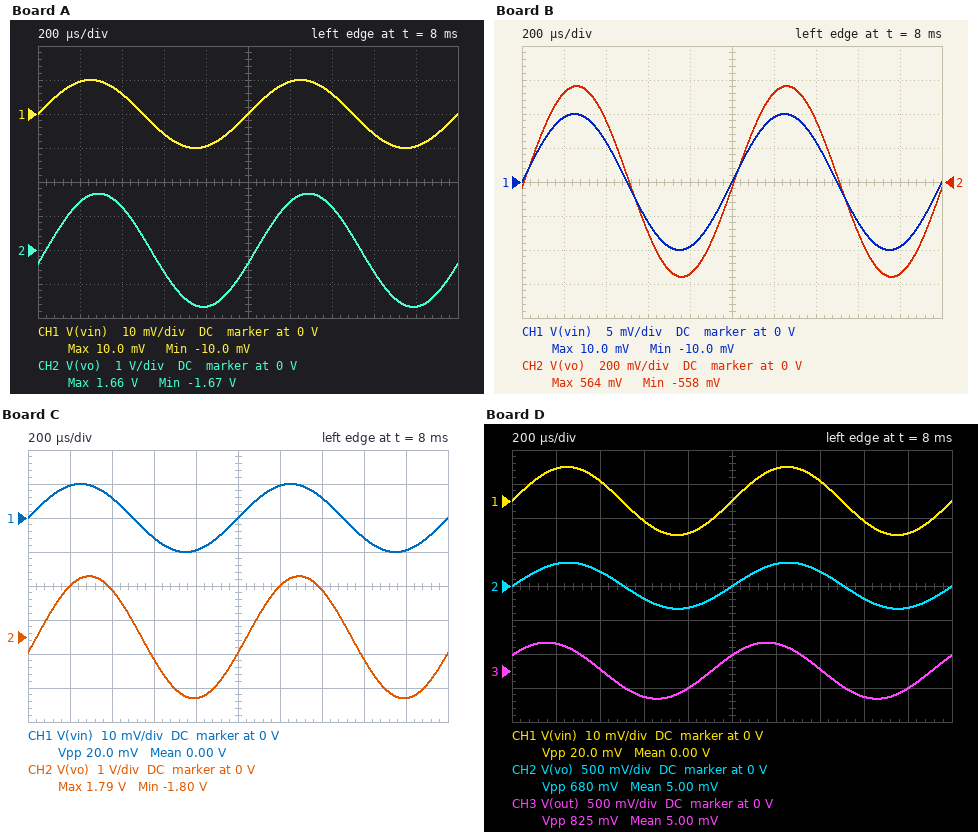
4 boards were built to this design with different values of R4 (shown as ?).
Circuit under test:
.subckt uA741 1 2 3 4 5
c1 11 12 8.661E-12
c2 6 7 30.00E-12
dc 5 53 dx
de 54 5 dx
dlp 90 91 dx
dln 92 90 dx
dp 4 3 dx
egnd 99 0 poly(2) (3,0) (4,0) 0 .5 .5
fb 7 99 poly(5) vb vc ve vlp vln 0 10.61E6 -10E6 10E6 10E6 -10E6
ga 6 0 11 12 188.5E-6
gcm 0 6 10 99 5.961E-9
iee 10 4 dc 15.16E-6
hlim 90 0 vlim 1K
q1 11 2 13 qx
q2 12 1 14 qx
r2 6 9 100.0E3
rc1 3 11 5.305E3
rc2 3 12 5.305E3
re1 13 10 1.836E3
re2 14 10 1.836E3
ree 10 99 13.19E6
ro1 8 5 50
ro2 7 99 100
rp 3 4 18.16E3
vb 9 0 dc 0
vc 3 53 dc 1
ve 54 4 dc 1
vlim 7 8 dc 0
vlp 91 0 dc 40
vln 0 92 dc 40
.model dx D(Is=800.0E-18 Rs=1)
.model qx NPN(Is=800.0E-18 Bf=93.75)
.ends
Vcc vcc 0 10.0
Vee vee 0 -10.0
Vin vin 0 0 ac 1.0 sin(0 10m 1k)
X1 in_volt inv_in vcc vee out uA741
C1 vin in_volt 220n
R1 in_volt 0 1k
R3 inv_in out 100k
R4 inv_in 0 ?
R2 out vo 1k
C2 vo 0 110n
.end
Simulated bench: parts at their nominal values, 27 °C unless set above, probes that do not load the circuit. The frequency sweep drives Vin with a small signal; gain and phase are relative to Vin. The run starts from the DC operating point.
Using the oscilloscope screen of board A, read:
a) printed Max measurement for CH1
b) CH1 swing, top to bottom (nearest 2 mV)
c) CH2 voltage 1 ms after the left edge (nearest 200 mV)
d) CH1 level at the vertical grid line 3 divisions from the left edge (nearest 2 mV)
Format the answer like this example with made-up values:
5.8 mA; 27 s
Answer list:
10.0 mV; 20 mV; -400 mV; -6 mV
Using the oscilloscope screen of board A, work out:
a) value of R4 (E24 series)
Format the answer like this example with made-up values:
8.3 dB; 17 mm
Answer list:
390 Ω
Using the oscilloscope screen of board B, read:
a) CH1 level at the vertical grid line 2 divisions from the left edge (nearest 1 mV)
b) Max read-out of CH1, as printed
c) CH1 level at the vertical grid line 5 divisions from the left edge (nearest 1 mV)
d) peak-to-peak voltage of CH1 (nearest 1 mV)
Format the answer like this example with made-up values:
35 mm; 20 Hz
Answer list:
6 mV; 10.0 mV; 0 V; 20 mV
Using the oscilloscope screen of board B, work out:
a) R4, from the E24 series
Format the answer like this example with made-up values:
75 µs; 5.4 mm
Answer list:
1.2 kΩ
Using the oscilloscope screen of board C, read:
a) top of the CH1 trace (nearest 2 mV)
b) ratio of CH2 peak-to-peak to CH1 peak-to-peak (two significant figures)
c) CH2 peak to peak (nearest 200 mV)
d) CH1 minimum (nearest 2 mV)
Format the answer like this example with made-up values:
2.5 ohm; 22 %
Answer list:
10 mV; 180; 3.6 V; -10 mV
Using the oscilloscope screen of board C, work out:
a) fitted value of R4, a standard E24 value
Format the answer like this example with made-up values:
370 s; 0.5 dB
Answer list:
360 Ω
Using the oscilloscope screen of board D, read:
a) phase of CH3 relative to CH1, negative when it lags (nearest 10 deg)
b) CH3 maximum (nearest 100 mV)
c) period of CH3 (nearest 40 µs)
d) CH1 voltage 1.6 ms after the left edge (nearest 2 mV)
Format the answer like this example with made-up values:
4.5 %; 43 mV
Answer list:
30 deg; 400 mV; 1.00 ms; -6 mV
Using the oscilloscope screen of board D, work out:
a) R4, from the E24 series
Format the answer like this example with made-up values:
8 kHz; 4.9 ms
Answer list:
2 kΩ
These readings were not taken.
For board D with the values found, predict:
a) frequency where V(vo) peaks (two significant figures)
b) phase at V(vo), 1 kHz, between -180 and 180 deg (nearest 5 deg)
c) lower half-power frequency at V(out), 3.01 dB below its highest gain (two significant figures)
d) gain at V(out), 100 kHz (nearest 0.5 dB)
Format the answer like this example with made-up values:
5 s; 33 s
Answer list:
1.0 kHz; 0 deg; 680 Hz; 19.5 dB
